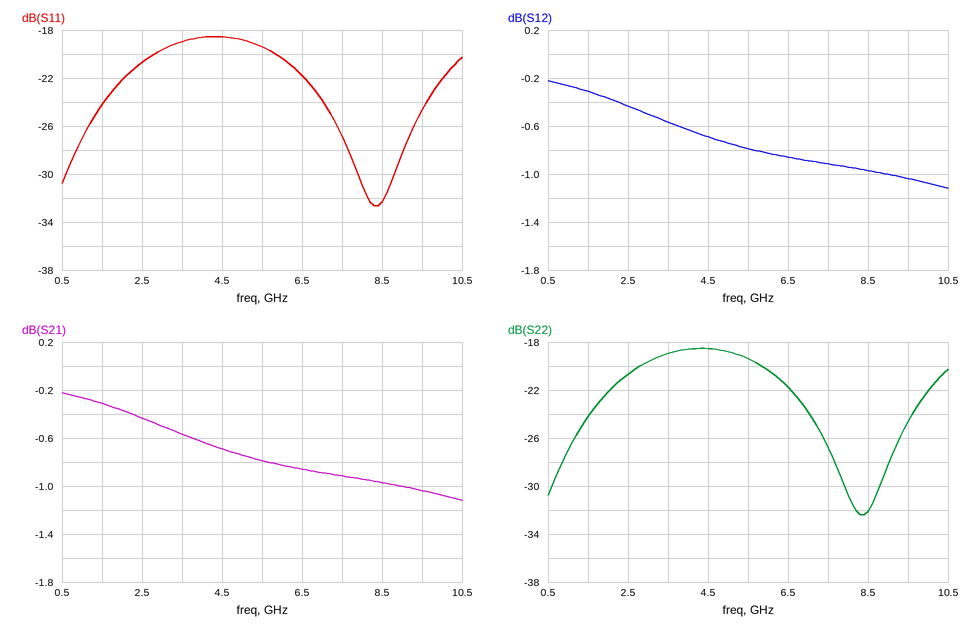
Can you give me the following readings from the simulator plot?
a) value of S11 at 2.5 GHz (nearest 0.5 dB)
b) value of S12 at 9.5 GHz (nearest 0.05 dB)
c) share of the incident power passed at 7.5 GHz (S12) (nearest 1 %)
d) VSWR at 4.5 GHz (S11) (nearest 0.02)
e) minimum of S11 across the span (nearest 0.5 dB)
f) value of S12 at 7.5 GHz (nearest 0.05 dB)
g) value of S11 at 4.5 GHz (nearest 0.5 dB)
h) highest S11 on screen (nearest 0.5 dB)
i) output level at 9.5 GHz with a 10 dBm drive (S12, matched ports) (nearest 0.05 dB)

-20.5 dB
-1.05 dB
81 %
1.26
-32.5 dB
-0.90 dB
-18.5 dB
-18.5 dB
8.95 dBm
